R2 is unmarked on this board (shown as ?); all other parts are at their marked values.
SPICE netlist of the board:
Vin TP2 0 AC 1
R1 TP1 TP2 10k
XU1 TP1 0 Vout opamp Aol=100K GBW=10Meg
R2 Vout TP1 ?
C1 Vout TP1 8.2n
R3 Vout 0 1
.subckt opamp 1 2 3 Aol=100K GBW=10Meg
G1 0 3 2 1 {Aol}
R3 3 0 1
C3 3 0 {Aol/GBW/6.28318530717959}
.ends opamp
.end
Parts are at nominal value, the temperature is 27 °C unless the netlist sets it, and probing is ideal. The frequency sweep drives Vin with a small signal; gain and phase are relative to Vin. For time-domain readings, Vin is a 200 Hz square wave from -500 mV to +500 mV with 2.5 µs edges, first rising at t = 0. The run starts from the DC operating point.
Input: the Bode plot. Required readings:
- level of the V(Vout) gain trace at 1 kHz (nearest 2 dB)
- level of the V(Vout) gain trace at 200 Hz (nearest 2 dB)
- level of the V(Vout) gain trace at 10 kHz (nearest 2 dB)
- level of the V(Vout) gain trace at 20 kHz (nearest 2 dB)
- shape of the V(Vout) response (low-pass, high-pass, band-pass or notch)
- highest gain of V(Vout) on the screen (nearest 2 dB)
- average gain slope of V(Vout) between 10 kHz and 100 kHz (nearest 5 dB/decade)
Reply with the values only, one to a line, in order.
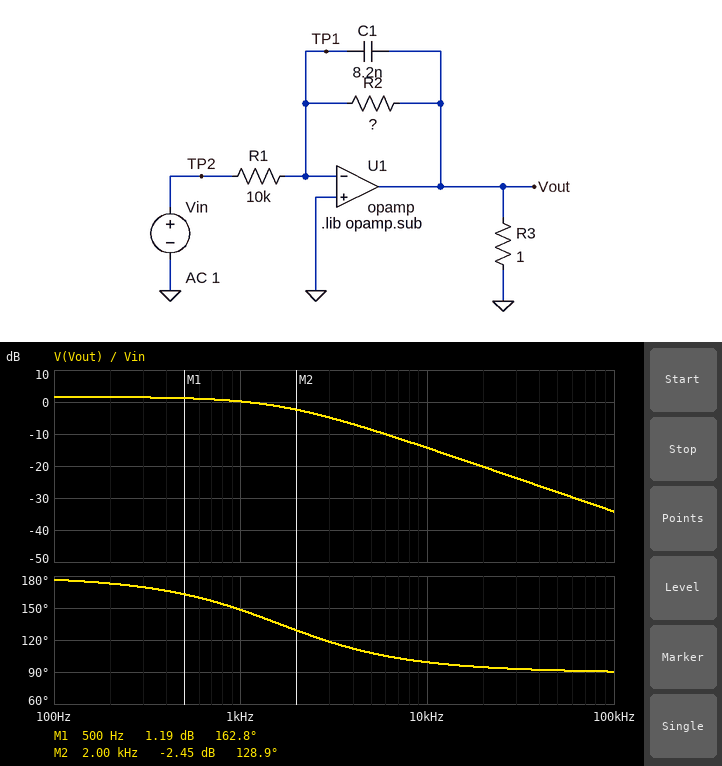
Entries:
0 dB
2 dB
-14 dB
-20 dB
low-pass
2 dB
-20 dB/decade
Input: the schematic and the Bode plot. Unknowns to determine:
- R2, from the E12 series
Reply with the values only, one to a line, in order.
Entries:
12 kΩ
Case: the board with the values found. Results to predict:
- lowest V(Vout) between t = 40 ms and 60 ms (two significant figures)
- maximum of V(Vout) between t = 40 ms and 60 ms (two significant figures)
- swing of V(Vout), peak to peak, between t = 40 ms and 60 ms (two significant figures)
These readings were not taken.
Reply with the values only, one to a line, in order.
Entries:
-600 mV
600 mV
1.2 V
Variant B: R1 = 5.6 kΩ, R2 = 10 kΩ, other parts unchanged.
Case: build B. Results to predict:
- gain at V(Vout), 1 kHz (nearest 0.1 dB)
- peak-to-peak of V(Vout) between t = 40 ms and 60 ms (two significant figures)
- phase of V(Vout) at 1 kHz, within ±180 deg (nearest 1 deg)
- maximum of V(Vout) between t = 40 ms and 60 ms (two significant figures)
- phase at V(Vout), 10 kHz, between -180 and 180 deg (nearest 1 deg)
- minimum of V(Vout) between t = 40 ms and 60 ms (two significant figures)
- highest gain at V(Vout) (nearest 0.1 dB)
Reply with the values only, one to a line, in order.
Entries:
4.0 dB
1.8 V
153 deg
890 mV
101 deg
-890 mV
5.0 dB
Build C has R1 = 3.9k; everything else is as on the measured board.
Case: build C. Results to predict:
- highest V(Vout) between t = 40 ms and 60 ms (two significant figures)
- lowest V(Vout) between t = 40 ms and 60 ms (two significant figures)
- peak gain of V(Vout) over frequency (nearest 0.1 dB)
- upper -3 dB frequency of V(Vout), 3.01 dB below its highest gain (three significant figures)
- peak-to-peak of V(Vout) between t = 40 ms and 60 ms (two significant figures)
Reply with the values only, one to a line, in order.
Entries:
1.5 V
-1.5 V
9.8 dB
1.62 kHz
3.1 V
